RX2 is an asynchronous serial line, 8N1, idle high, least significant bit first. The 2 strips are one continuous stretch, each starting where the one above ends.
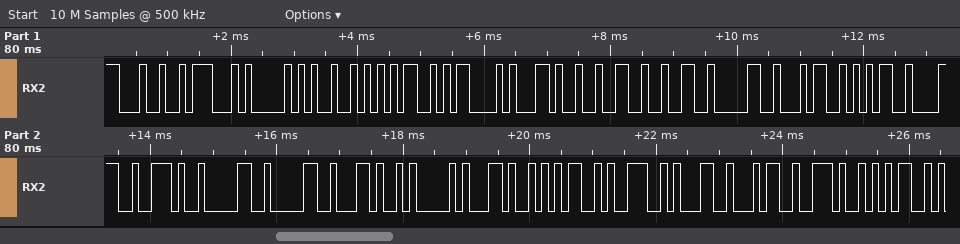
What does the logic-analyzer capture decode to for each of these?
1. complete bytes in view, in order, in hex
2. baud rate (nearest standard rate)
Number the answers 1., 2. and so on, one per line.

1. 24 47 50 52 4D 43 2C 32 32 30 34 35 38 2E 30 30 2C 41 2C 35 39 31 34 2E 35
2. 9600 baud
